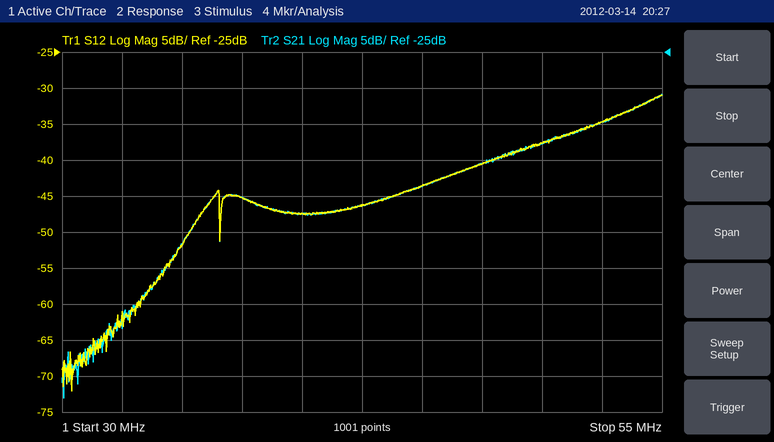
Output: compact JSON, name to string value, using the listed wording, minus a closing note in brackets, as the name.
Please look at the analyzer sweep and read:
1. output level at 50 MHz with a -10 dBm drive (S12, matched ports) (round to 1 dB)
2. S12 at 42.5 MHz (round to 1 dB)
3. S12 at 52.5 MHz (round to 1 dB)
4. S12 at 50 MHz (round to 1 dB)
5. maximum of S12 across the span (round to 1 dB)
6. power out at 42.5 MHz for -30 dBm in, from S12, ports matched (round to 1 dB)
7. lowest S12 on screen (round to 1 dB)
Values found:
{"output level at 50 MHz with a -10 dBm drive (S12, matched ports)": "-48 dBm", "S12 at 42.5 MHz": "-46 dB", "S12 at 52.5 MHz": "-35 dB", "S12 at 50 MHz": "-38 dB", "maximum of S12 across the span": "-31 dB", "power out at 42.5 MHz for -30 dBm in, from S12, ports matched": "-76 dBm", "lowest S12 on screen": "-72 dB"}
